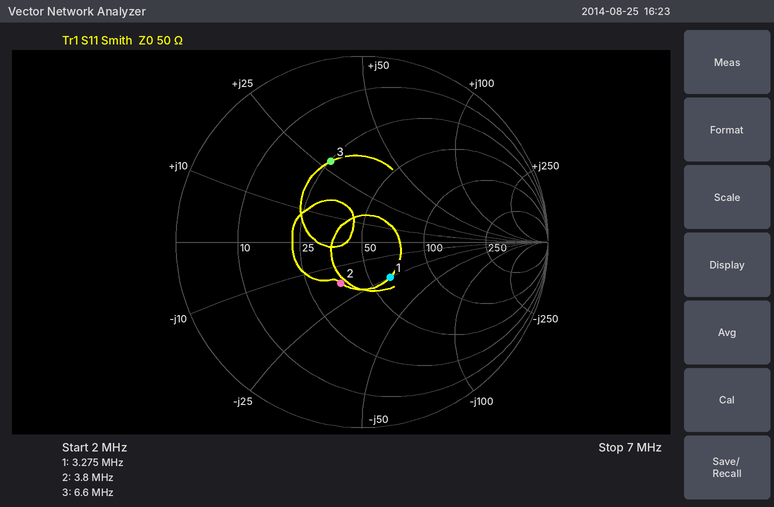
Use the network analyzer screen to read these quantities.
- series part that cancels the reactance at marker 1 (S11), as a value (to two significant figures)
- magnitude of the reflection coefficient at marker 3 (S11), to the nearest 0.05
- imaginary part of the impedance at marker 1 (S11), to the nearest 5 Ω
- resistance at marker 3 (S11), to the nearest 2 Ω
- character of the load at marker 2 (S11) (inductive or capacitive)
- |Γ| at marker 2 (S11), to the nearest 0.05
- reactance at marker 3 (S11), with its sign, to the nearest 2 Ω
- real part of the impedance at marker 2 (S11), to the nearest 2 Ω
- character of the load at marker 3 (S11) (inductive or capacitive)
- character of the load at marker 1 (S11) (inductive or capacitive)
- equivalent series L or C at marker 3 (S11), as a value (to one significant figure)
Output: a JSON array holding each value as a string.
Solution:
["1.2 µH", "0.45", "-25 Ω", "26 Ω", "capacitive", "0.25", "+28 Ω", "36 Ω", "inductive", "capacitive", "700 nH"]
